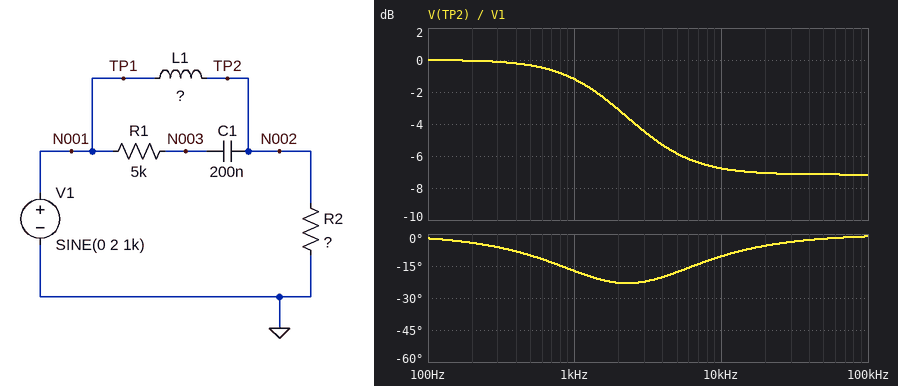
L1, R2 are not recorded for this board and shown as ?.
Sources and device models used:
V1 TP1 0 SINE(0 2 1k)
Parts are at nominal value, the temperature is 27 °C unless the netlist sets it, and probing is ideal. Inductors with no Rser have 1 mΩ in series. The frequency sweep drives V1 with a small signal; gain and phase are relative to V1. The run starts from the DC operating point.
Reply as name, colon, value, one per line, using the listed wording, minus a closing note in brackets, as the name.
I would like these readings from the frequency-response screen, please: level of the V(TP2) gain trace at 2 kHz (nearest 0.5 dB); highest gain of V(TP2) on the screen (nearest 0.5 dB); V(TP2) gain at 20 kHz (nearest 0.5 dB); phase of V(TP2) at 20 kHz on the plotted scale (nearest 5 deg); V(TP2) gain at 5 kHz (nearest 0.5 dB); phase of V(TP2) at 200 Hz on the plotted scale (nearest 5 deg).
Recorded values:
level of the V(TP2) gain trace at 2 kHz: -3.0 dB
highest gain of V(TP2) on the screen: 0 dB
V(TP2) gain at 20 kHz: -7.0 dB
phase of V(TP2) at 20 kHz on the plotted scale: -5 deg
V(TP2) gain at 5 kHz: -6.0 dB
phase of V(TP2) at 200 Hz on the plotted scale: -5 deg
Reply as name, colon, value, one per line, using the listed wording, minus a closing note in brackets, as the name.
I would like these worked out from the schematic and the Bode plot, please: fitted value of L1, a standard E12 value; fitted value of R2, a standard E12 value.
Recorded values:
fitted value of L1, a standard E12 value: 220 mH
fitted value of R2, a standard E12 value: 3.9 kΩ
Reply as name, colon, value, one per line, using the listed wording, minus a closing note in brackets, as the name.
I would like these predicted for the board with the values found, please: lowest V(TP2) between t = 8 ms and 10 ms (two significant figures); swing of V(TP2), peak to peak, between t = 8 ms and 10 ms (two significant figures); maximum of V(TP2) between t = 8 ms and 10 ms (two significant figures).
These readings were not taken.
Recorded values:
lowest V(TP2) between t = 8 ms and 10 ms: -1.7 V
swing of V(TP2), peak to peak, between t = 8 ms and 10 ms: 3.5 V
maximum of V(TP2) between t = 8 ms and 10 ms: 1.7 V
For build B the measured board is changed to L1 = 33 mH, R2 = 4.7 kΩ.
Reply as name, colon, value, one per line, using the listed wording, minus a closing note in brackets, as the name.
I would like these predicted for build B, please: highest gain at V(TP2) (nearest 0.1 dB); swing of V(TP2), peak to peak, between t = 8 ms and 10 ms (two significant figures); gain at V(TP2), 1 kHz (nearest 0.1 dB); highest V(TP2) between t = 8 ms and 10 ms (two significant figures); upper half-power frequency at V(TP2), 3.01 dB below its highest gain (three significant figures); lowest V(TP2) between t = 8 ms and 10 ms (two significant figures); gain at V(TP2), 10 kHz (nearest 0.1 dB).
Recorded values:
highest gain at V(TP2): 0 dB
swing of V(TP2), peak to peak, between t = 8 ms and 10 ms: 4.0 V
gain at V(TP2), 1 kHz: 0 dB
highest V(TP2) between t = 8 ms and 10 ms: 2.0 V
upper half-power frequency at V(TP2), 3.01 dB below its highest gain: 15.9 kHz
lowest V(TP2) between t = 8 ms and 10 ms: -2.0 V
gain at V(TP2), 10 kHz: -1.7 dB
